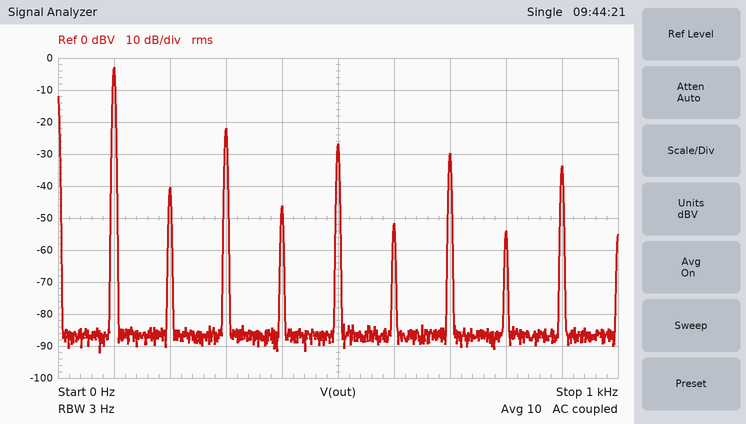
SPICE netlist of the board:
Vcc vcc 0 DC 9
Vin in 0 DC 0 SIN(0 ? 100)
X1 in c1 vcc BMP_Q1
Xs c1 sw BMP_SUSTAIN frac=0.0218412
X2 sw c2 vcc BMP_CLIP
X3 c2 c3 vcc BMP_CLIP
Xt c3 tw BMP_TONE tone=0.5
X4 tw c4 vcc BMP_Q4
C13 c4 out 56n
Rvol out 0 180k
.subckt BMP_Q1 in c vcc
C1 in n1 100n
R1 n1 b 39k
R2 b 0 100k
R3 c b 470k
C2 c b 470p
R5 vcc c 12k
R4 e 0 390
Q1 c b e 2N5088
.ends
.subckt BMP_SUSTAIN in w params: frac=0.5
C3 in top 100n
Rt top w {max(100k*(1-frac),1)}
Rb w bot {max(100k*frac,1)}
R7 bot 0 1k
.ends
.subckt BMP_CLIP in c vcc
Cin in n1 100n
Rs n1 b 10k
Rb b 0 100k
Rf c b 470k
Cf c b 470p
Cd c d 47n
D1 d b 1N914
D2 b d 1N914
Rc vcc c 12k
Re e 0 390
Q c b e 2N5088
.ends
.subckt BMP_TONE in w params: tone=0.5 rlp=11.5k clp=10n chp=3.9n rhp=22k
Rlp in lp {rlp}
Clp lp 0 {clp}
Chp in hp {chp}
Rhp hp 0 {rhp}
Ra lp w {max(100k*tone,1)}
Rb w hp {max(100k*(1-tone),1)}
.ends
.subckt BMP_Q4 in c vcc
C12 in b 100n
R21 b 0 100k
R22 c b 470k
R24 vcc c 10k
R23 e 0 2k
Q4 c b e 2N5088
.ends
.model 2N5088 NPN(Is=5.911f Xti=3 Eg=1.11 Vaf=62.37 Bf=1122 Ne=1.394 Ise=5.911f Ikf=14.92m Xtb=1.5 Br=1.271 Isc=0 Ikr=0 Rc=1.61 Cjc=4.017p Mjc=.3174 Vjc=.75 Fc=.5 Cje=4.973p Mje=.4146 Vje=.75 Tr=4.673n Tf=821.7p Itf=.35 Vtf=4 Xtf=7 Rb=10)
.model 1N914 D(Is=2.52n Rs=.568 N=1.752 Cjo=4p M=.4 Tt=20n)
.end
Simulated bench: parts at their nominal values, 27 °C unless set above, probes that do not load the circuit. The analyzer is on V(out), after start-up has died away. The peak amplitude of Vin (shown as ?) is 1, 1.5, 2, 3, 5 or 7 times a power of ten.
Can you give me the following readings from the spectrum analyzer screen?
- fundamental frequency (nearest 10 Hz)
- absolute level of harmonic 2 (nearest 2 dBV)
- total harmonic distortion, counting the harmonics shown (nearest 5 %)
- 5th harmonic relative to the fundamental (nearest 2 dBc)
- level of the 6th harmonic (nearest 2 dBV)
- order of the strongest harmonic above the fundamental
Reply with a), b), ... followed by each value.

a) 100 Hz
b) -40 dBV
c) 15 %
d) -24 dBc
e) -52 dBV
f) 3
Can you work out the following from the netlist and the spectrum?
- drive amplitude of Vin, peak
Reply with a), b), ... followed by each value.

a) 500 mV
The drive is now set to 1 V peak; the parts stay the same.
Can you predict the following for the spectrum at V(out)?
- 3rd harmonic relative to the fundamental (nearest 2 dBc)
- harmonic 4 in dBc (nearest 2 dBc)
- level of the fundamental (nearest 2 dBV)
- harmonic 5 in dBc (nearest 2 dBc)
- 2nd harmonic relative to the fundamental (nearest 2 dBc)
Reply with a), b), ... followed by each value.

a) -22 dBc
b) -28 dBc
c) -2 dBV
d) -26 dBc
e) -24 dBc
